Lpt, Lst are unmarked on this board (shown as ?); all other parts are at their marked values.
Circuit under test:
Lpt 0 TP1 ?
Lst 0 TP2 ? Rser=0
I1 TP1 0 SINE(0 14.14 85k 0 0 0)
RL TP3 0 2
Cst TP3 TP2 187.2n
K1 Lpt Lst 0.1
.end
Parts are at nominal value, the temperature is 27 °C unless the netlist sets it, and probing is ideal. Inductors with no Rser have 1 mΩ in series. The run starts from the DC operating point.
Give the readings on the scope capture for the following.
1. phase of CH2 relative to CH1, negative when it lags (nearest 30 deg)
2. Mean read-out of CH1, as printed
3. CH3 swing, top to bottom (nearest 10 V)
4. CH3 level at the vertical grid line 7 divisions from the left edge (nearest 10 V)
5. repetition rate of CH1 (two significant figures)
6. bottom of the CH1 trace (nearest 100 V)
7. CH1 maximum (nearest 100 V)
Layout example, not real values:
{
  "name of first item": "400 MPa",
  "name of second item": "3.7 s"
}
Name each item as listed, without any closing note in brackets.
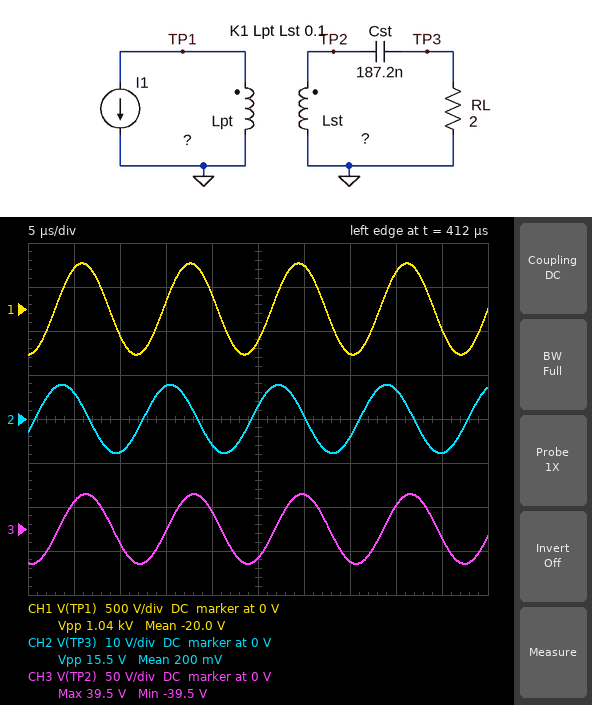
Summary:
{
  "phase of CH2 relative to CH1, negative when it lags": "60 deg",
  "Mean read-out of CH1, as printed": "-20.0 V",
  "CH3 swing, top to bottom": "80 V",
  "CH3 level at the vertical grid line 7 divisions from the left edge": "-40 V",
  "repetition rate of CH1": "85 kHz",
  "bottom of the CH1 trace": "-500 V",
  "CH1 maximum": "500 V"
}
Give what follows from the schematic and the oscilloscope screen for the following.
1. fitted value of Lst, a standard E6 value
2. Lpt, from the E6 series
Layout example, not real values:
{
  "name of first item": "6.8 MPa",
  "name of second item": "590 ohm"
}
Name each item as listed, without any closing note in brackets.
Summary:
{
  "fitted value of Lst, a standard E6 value": "10 µH",
  "Lpt, from the E6 series": "68 µH"
}
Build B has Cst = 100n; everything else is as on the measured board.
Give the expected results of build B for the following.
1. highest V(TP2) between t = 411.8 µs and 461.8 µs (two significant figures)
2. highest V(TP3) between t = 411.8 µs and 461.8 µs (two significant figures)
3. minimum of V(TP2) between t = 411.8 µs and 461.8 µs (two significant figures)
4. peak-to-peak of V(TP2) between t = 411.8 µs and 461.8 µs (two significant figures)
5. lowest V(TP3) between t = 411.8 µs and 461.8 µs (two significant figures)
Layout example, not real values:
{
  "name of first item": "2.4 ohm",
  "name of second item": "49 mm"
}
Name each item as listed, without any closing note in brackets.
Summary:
{
  "highest V(TP2) between t = 411.8 µs and 461.8 µs": "27 V",
  "highest V(TP3) between t = 411.8 µs and 461.8 µs": "2.9 V",
  "minimum of V(TP2) between t = 411.8 µs and 461.8 µs": "-27 V",
  "peak-to-peak of V(TP2) between t = 411.8 µs and 461.8 µs": "55 V",
  "lowest V(TP3) between t = 411.8 µs and 461.8 µs": "-2.9 V"
}
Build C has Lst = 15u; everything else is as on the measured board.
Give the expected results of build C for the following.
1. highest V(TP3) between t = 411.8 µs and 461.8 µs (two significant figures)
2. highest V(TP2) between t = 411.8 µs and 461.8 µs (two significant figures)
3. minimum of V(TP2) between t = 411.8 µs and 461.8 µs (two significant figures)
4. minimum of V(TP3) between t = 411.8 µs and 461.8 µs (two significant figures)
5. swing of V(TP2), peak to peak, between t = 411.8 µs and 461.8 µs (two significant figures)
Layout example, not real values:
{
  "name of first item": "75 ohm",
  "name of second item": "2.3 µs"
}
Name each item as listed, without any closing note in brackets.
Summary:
{
  "highest V(TP3) between t = 411.8 µs and 461.8 µs": "17 V",
  "highest V(TP2) between t = 411.8 µs and 461.8 µs": "87 V",
  "minimum of V(TP2) between t = 411.8 µs and 461.8 µs": "-87 V",
  "minimum of V(TP3) between t = 411.8 µs and 461.8 µs": "-17 V",
  "swing of V(TP2), peak to peak, between t = 411.8 µs and 461.8 µs": "170 V"
}
